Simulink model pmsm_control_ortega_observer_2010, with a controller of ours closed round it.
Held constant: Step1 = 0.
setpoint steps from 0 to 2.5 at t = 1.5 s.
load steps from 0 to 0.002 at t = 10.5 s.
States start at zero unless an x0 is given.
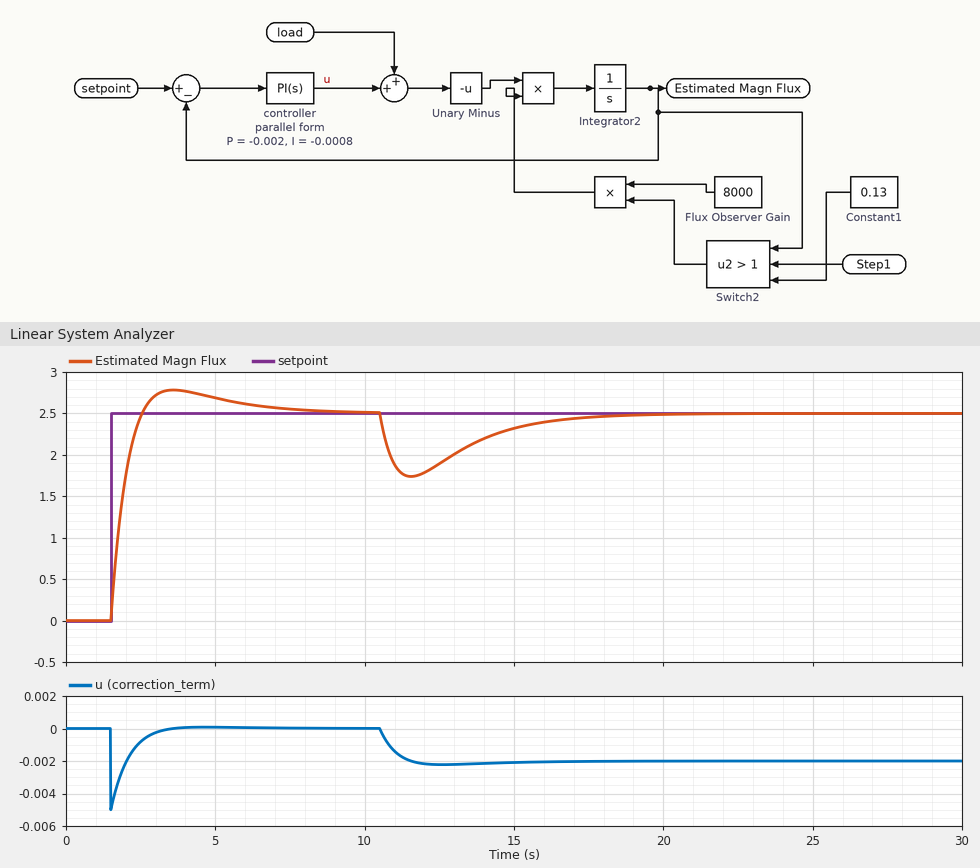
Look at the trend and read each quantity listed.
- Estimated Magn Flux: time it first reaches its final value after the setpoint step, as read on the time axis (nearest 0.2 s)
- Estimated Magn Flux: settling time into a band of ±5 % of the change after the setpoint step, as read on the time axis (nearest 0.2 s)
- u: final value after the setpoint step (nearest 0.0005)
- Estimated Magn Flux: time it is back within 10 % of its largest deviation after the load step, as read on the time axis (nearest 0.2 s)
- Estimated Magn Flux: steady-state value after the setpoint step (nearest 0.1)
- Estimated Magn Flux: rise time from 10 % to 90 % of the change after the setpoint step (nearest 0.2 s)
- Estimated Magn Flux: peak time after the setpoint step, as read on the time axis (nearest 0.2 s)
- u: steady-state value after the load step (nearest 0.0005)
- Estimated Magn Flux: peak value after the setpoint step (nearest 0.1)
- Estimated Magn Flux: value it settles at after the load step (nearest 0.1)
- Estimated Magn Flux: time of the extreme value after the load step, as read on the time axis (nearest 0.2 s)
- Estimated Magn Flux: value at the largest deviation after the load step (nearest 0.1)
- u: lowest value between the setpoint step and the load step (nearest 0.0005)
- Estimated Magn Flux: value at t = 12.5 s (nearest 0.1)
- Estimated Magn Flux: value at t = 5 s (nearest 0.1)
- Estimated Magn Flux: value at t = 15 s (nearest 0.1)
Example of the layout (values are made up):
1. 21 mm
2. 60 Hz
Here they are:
1. 2.6 s
2. 5.8 s
3. 0.0000
4. 16.6 s
5. 2.5
6. 0.8 s
7. 3.6 s
8. -0.0020
9. 2.8
10. 2.5
11. 11.6 s
12. 1.7
13. -0.0050
14. 1.9
15. 2.7
16. 2.3
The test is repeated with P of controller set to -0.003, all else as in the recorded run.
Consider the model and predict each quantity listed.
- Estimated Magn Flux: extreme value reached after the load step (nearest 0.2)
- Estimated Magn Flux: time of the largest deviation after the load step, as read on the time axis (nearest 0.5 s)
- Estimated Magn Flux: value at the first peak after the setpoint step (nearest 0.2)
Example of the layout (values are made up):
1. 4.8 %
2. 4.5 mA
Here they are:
1. 2.0
2. 11.5 s
3. 2.6
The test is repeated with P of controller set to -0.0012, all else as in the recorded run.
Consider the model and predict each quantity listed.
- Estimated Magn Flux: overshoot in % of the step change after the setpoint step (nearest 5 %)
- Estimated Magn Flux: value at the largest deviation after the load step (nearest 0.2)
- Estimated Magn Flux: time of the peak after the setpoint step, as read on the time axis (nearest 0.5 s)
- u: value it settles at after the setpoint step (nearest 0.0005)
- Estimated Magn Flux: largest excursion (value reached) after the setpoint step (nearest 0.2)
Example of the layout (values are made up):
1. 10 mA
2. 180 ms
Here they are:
1. 20 %
2. 1.4
3. 4.0 s
4. 0.0000
5. 3.0
